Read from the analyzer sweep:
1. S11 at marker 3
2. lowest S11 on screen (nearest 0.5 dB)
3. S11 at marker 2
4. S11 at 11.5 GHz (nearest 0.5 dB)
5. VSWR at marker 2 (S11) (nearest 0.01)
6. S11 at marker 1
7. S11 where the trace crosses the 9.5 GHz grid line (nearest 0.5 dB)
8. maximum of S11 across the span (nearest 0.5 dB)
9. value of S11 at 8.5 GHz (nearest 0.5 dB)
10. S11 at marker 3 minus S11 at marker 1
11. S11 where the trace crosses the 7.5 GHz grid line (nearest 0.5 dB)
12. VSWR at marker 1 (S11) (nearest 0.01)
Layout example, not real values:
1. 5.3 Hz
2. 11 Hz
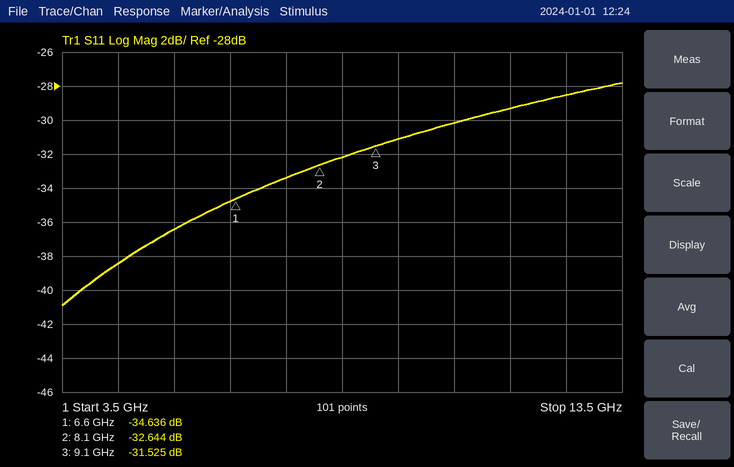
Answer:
1. -31.525 dB
2. -41.0 dB
3. -32.644 dB
4. -29.5 dB
5. 1.05
6. -34.636 dB
7. -31.0 dB
8. -28.0 dB
9. -32.0 dB
10. 3.111 dB
11. -33.5 dB
12. 1.04
